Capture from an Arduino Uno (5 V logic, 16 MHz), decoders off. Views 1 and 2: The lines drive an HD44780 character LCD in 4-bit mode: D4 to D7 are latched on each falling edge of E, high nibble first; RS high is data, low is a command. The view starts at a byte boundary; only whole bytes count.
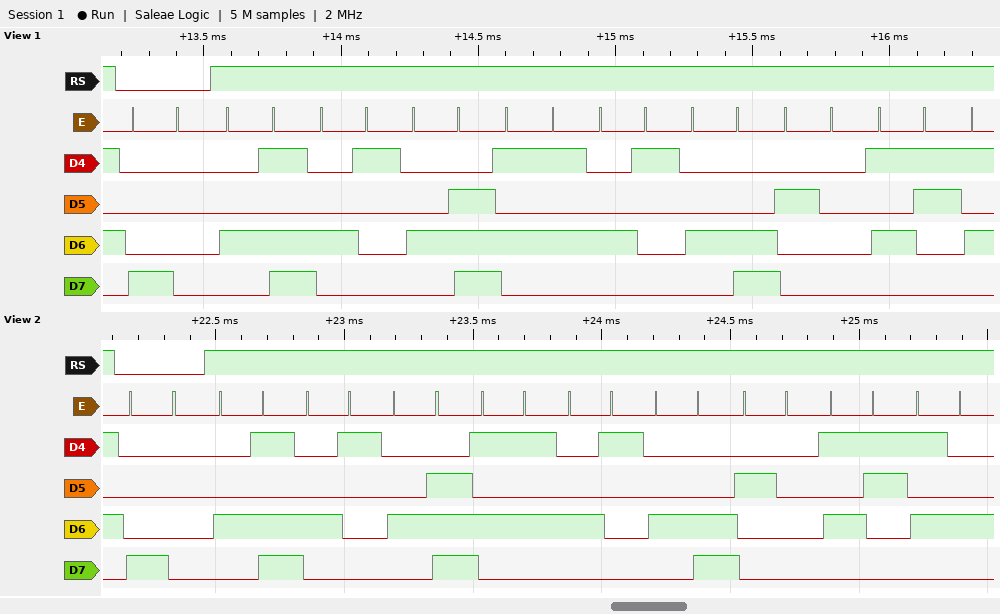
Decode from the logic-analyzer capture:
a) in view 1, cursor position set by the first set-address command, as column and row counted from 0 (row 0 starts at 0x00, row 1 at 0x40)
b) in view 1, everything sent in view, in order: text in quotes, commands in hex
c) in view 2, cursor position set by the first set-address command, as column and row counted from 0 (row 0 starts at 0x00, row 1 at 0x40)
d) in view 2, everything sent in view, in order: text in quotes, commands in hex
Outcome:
column 0, row 0
0x80 "MANUAL S"
column 0, row 0
0x80 "MANUAL ST"
